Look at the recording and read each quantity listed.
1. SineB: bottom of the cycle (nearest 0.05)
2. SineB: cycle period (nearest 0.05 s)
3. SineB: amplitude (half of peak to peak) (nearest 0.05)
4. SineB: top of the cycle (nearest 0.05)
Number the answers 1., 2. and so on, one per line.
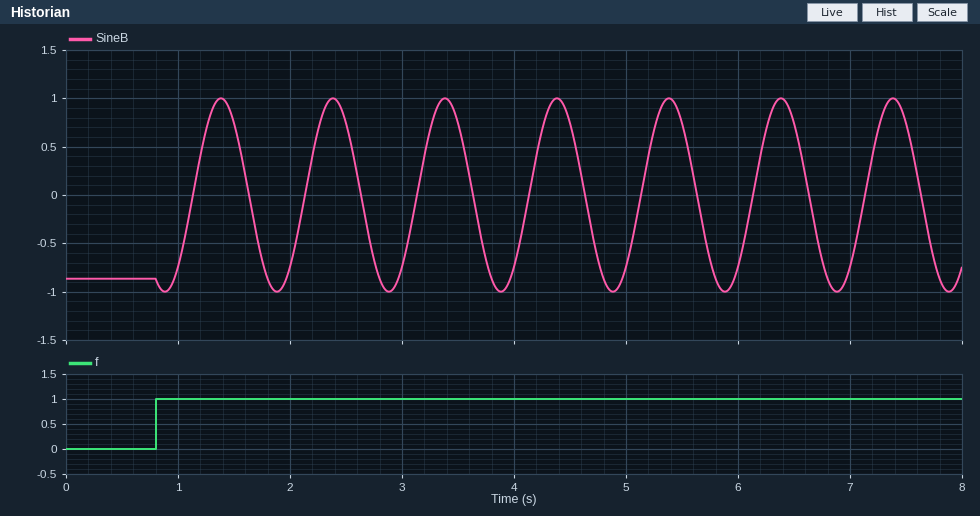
1. -1.00
2. 1.00 s
3. 1.00
4. 1.00
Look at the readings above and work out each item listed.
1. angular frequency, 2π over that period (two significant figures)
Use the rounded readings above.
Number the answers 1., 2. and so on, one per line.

1. 6.3 rad/s
